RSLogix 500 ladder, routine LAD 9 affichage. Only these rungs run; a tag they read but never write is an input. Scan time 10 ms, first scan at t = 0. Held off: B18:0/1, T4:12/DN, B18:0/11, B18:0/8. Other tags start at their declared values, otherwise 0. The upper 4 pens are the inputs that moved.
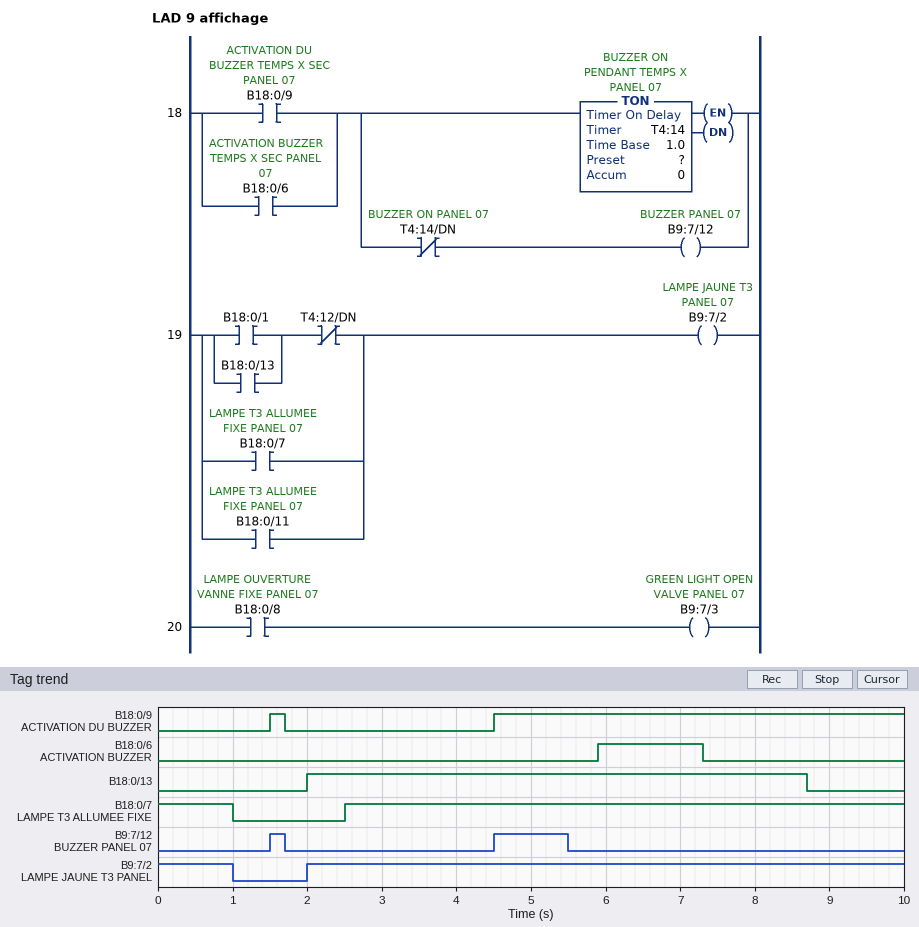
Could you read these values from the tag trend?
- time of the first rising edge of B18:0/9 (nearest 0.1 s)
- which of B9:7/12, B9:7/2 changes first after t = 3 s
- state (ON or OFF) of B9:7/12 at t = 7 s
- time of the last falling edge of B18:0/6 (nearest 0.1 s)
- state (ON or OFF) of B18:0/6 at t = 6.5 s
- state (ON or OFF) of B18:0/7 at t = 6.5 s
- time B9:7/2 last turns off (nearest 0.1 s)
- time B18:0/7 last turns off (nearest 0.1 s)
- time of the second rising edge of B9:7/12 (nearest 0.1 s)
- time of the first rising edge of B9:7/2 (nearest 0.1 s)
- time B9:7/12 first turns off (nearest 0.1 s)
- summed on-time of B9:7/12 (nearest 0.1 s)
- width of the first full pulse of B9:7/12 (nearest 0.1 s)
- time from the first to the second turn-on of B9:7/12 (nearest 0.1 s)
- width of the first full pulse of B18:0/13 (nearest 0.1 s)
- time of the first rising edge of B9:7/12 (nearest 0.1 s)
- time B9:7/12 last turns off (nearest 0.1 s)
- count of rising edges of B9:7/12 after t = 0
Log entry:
1.5 s
B9:7/12
OFF
7.3 s
ON
ON
1.0 s
1.0 s
4.5 s
2.0 s
1.7 s
1.2 s
0.2 s
3.0 s
6.7 s
1.5 s
5.5 s
2
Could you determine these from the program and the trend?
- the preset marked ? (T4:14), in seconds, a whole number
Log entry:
1 s
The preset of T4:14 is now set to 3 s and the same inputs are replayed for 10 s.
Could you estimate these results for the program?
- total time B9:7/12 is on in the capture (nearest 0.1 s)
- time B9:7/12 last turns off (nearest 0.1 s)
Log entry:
3.2 s
7.5 s
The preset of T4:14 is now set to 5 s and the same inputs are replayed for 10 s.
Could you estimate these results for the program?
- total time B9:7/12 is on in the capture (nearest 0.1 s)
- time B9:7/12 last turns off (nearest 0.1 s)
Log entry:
5.2 s
9.5 s
